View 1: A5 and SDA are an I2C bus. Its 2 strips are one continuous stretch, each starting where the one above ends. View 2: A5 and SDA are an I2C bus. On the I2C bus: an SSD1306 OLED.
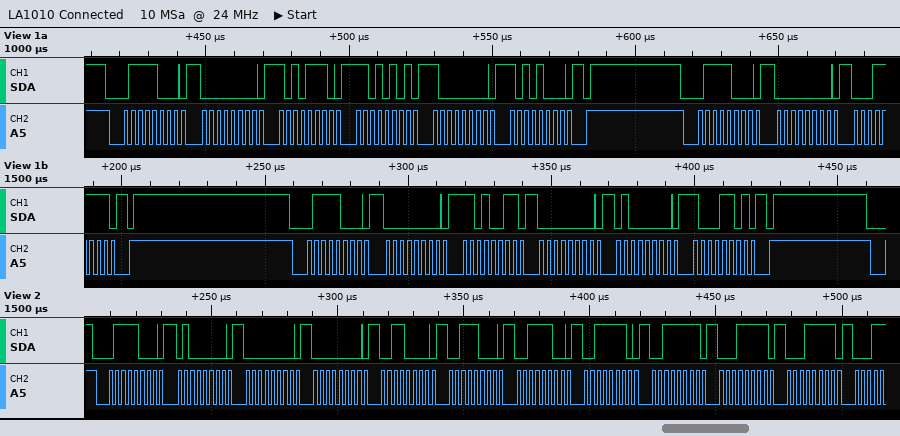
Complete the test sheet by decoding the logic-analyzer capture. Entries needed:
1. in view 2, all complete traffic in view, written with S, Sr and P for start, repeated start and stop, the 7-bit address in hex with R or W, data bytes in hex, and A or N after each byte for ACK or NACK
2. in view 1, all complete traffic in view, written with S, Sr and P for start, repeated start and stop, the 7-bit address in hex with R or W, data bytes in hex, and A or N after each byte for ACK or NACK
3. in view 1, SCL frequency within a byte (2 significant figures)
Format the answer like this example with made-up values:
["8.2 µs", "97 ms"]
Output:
["S 3CW A 40 A 00 A 00 A 30 A 38 A 3C A 3E A 3F A 1F A 1F A", "S 3CW A 00 A AE A D5 A 80 A A8 A P S 3CW A 00 A 1F A P S 3CW A 00 A D3 A 00 A 40 A 8D A P", "400 kHz"]
